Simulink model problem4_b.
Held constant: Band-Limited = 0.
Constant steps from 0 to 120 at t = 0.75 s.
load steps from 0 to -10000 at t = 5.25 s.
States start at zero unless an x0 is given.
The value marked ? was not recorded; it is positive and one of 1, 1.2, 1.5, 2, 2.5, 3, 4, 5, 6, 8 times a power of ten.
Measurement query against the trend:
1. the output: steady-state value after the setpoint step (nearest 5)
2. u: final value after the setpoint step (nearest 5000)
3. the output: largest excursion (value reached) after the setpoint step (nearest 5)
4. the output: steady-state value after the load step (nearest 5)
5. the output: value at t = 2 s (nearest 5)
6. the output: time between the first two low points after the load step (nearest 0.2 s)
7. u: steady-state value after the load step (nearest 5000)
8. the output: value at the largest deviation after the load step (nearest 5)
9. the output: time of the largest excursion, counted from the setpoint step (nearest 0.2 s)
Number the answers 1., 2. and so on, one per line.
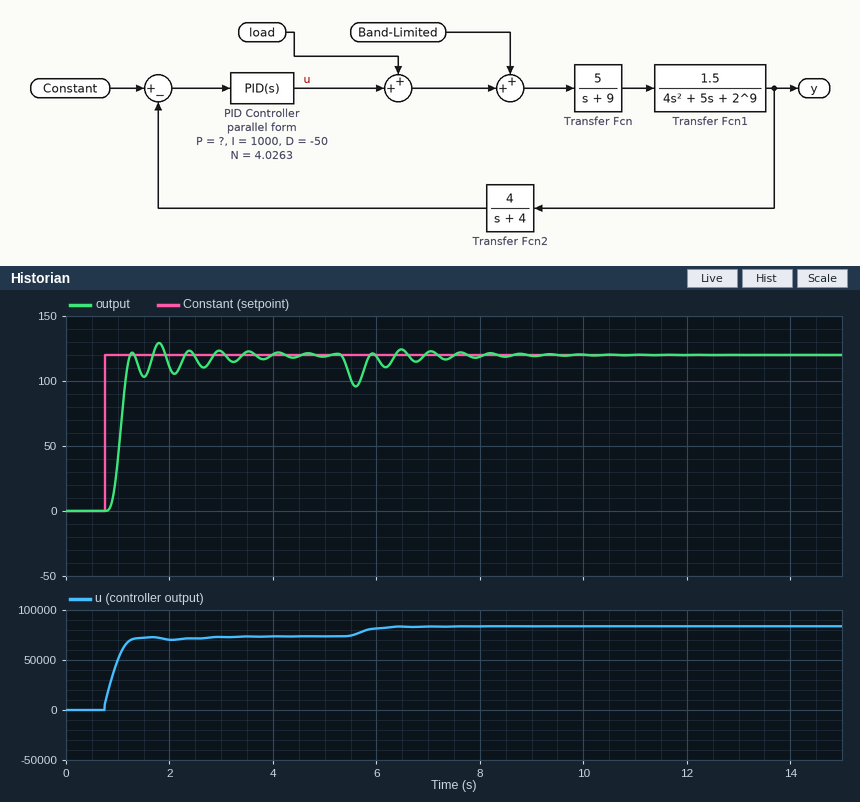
1. 120
2. 75000
3. 130
4. 120
5. 110
6. 0.6 s
7. 85000
8. 95
9. 1.0 s
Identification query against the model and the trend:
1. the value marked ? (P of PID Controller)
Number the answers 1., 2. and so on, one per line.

1. 250
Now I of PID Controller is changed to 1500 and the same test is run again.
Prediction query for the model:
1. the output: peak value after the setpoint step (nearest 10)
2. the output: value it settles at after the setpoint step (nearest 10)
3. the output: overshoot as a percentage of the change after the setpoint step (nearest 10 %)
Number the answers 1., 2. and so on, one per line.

1. 160
2. 120
3. 30 %
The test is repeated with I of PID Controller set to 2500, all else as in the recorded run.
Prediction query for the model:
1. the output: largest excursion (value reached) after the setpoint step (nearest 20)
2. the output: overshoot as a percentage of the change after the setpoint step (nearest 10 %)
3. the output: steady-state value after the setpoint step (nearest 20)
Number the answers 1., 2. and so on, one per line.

1. 240
2. 90 %
3. 120
